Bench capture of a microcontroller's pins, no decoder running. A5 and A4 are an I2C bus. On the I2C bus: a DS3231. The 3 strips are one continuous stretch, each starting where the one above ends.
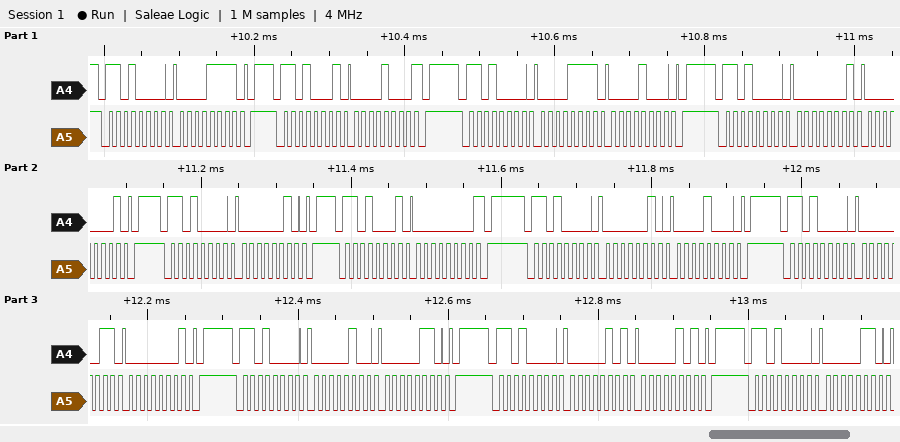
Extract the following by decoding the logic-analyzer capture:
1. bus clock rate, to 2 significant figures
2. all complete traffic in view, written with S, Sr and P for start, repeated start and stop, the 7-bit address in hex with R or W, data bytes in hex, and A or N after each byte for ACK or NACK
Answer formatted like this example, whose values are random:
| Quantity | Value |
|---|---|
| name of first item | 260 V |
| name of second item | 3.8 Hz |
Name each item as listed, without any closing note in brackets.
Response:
| Quantity | Value |
|---|---|
| bus clock rate, to 2 significant figures | 100 kHz |
| all complete traffic in view, written with S, Sr and P for start, repeated start and stop, the 7-bit address in hex with R or W, data bytes in hex, and A or N after each byte for ACK or NACK | S 68W A 0F A P S 68R A 08 N P S 68W A 0F A 08 A P S 68W A 01 A 01 A P S 68W A 02 A P S 68R A 00 N P S 68W A 02 A 08 A P S 68W A 03 A 01 A P S 68W A 04 A 06 A P S 68W A 05 A 05 A P S 68W A 06 A |
